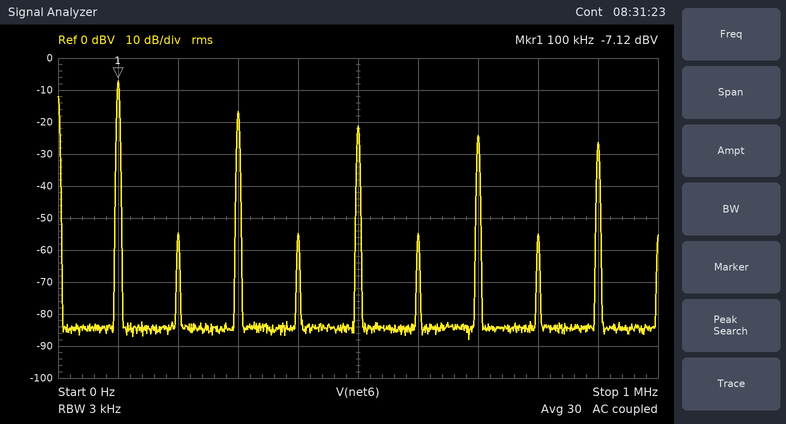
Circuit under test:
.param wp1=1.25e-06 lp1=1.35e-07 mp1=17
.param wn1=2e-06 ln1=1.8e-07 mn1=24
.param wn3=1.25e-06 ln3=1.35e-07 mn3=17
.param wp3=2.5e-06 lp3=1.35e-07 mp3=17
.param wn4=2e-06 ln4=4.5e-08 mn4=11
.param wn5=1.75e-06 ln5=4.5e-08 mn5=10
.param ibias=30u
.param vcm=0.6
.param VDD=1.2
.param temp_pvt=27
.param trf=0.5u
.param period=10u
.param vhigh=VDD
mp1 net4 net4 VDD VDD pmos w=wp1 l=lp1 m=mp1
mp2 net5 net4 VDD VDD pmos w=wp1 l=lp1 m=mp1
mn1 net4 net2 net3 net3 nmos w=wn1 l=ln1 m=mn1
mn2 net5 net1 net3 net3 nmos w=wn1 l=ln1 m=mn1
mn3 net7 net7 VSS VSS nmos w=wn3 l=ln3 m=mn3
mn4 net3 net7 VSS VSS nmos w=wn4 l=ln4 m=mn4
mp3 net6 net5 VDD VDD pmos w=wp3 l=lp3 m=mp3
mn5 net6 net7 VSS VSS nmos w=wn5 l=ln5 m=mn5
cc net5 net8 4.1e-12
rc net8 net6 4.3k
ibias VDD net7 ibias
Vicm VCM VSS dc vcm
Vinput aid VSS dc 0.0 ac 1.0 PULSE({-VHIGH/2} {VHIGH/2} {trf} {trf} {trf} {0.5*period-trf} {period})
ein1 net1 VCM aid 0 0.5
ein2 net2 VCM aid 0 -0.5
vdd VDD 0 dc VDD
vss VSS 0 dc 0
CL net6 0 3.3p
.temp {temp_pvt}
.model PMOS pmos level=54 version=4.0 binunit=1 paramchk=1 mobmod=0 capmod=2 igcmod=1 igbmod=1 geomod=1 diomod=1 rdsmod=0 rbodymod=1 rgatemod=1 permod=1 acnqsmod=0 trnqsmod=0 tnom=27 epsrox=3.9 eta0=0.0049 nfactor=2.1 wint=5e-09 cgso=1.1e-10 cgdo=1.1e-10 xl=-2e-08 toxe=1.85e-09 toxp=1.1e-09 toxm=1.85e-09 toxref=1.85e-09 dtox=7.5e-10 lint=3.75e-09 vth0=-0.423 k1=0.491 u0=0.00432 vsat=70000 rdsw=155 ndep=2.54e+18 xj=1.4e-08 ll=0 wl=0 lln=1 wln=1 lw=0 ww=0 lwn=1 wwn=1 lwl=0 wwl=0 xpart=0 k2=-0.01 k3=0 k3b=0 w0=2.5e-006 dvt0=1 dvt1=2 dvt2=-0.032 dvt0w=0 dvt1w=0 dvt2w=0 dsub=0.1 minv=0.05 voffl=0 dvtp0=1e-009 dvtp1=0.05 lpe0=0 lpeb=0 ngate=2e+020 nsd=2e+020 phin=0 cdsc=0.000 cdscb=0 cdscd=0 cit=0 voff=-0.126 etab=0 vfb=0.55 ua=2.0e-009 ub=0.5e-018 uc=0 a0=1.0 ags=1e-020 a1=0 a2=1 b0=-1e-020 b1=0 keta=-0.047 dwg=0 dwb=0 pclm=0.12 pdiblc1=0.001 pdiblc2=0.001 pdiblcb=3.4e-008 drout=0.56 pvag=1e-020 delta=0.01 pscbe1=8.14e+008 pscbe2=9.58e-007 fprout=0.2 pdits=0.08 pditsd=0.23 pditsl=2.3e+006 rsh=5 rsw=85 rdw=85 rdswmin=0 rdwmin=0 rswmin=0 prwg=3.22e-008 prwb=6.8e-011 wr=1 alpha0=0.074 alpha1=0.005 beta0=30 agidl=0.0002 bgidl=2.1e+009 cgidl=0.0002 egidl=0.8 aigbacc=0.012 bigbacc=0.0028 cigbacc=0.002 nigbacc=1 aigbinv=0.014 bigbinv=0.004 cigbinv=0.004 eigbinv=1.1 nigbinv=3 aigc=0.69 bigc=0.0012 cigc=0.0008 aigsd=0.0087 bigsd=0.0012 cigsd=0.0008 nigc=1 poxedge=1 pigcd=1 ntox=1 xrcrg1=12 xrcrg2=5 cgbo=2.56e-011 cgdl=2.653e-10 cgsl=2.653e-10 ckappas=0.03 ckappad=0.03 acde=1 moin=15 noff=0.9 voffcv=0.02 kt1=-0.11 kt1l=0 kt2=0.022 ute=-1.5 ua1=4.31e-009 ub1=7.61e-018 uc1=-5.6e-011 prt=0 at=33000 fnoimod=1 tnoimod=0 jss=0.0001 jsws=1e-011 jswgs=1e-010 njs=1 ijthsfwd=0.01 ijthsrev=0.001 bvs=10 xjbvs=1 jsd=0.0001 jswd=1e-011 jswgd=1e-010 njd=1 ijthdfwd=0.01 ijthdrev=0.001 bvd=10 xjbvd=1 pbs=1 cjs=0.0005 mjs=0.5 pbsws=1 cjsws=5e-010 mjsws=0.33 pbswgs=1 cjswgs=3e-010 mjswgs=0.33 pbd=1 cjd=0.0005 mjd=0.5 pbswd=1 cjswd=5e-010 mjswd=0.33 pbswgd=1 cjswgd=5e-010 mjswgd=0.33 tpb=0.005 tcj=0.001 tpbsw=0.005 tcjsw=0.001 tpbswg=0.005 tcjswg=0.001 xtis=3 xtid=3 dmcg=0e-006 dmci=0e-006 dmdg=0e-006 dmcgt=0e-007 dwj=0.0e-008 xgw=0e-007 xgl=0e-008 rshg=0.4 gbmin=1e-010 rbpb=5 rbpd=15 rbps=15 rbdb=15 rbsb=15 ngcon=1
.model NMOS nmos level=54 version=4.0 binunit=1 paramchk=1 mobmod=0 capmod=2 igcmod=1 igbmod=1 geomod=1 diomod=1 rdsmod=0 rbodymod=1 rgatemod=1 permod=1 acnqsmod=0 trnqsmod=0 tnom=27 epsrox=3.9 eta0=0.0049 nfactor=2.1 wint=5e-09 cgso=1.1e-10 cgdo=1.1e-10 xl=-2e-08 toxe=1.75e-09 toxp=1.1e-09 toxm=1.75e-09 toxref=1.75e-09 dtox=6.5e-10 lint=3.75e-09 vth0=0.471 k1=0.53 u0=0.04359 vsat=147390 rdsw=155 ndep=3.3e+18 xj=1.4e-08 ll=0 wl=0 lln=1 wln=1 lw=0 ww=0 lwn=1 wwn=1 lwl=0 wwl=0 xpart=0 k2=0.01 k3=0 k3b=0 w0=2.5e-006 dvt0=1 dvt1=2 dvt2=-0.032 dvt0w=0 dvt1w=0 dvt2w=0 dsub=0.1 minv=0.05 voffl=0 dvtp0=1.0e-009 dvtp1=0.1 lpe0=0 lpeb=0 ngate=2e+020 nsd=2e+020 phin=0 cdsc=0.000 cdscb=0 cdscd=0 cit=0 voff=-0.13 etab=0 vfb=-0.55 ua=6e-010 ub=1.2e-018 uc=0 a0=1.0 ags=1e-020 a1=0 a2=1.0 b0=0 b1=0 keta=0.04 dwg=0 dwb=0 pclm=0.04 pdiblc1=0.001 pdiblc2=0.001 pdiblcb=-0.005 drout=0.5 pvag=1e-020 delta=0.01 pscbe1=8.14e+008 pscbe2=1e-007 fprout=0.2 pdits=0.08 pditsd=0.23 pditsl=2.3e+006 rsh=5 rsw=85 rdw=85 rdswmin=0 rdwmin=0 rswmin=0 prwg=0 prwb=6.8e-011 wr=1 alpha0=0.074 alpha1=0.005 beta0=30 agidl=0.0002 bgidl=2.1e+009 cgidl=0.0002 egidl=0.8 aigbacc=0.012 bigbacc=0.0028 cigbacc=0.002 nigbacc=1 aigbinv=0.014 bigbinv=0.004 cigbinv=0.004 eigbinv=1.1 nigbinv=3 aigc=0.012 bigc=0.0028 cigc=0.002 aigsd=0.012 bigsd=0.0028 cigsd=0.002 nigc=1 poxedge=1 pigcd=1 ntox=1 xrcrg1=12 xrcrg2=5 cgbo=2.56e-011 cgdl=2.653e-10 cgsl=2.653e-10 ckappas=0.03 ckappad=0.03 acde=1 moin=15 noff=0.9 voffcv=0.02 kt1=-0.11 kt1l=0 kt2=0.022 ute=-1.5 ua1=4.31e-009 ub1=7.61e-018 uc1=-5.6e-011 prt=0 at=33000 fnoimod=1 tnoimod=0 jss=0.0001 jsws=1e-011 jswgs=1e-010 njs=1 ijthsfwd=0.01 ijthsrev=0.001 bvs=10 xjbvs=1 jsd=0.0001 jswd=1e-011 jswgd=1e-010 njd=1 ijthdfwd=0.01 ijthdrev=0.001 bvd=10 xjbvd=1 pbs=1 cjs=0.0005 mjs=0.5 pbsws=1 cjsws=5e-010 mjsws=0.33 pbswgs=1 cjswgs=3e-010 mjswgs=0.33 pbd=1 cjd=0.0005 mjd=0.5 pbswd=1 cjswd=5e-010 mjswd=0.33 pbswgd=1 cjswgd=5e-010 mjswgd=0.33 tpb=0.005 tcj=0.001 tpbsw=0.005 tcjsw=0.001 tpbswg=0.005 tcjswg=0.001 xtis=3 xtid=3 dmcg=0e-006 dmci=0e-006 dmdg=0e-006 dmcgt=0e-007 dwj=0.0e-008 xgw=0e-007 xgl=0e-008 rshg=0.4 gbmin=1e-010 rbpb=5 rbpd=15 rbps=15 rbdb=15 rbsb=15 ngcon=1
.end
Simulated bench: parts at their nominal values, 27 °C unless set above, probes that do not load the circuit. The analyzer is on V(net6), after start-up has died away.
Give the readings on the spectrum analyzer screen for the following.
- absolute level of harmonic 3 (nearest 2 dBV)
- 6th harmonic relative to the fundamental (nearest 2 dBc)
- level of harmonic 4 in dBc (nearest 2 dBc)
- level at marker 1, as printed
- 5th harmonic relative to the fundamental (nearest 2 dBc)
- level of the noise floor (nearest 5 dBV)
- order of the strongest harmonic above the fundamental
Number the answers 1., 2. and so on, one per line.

1. -16 dBV
2. -48 dBc
3. -48 dBc
4. -7.12 dBV
5. -14 dBc
6. -85 dBV
7. 3
